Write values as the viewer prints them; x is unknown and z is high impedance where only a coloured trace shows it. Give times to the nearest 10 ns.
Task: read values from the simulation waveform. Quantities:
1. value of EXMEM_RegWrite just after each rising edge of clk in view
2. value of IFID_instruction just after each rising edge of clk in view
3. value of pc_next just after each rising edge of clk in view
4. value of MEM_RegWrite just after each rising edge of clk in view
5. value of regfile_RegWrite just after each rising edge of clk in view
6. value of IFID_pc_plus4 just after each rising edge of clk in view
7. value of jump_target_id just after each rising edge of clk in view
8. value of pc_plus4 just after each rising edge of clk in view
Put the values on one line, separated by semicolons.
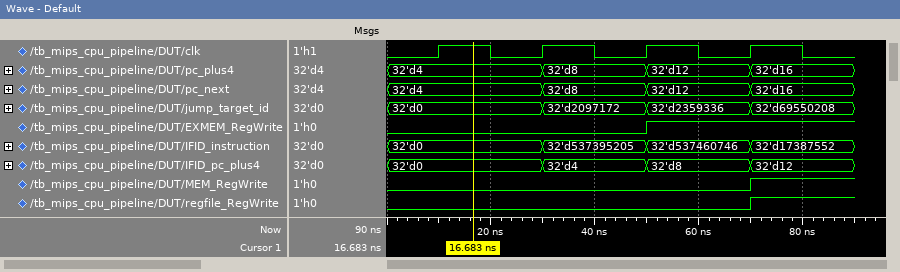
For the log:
0 0 1 1; 32'd0, 32'd537395205, 32'd537460746, 32'd17387552; 32'd4, 32'd8, 32'd12, 32'd16; 0 0 0 1; 0 0 0 1; 32'd0, 32'd4, 32'd8, 32'd12; 32'd0, 32'd2097172, 32'd2359336, 32'd69550208; 32'd4, 32'd8, 32'd12, 32'd16
